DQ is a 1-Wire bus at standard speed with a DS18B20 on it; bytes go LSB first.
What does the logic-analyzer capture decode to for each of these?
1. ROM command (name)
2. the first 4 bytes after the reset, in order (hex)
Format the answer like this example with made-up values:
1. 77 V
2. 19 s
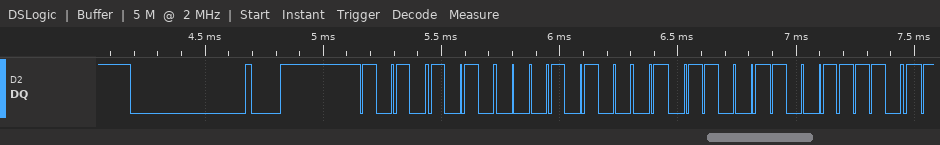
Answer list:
1. Match ROM
2. 55 28 9A 79
